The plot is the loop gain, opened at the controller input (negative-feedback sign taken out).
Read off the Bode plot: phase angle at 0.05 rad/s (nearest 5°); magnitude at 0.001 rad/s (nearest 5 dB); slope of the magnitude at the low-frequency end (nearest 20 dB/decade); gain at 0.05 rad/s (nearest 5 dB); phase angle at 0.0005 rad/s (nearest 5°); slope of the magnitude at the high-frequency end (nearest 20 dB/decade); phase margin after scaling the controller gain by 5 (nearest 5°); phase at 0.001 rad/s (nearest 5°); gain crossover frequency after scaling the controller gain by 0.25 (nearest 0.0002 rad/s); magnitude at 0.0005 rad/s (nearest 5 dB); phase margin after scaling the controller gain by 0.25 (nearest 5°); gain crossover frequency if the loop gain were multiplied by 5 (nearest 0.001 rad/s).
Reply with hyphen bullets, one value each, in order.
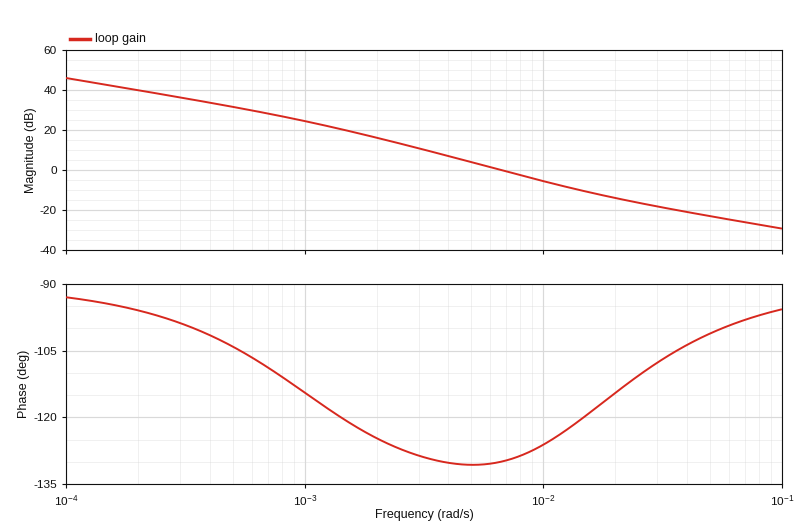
- -100°
- 25 dB
- -20 dB/decade
- -25 dB
- -105°
- -20 dB/decade
- 65°
- -115°
- 0.0028 rad/s
- 30 dB
- 50°
- 0.020 rad/s
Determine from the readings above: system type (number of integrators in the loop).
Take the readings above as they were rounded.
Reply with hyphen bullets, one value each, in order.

- 1
